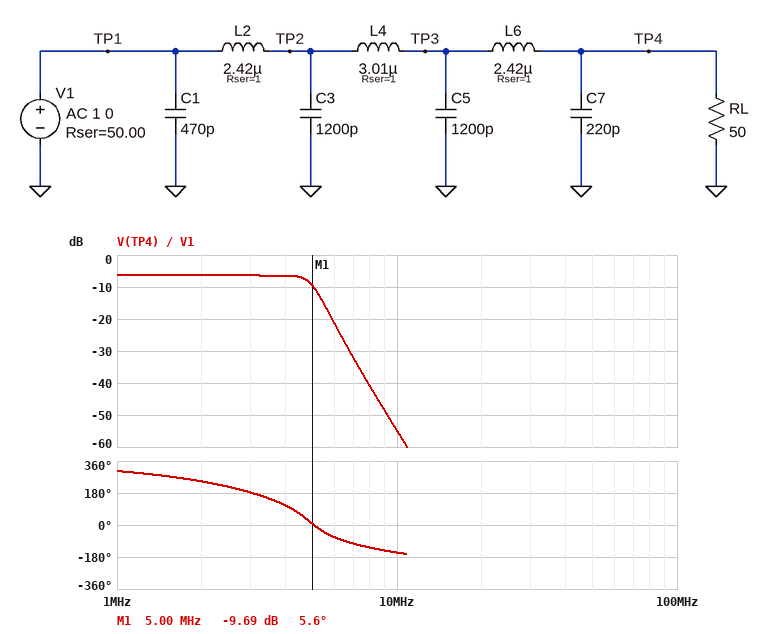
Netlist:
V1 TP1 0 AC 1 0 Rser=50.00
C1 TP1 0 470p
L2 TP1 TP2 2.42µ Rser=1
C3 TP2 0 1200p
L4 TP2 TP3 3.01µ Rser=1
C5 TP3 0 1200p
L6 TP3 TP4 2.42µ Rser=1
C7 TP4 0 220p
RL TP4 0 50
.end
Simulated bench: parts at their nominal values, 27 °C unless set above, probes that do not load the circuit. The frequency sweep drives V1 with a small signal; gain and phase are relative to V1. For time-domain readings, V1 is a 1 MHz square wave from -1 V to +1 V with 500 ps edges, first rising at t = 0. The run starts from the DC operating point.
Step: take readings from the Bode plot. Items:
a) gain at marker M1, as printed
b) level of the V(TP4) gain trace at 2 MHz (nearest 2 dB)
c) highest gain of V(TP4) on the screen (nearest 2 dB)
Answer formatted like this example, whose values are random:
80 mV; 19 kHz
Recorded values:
-9.69 dB; -6 dB; -6 dB
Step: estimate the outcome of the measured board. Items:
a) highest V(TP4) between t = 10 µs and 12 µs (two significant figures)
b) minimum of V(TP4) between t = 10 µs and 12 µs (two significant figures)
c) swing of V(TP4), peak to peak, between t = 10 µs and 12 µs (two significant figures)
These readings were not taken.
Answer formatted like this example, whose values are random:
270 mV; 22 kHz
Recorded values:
650 mV; -650 mV; 1.3 V
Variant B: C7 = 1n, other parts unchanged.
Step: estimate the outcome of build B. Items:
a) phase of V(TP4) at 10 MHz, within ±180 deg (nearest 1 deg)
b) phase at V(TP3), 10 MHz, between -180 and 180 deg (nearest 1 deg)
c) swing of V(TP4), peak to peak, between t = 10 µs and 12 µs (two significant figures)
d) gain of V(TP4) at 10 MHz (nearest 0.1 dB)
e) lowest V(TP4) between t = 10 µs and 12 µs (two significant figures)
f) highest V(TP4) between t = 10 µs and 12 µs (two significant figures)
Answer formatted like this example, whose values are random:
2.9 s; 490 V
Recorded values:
153 deg; -47 deg; 1.3 V; -63.8 dB; -670 mV; 670 mV
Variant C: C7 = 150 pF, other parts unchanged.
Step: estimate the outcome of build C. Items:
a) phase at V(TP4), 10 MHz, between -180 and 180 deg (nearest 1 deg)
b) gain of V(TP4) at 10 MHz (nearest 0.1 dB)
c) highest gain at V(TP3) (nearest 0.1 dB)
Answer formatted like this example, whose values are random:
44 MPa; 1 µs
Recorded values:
-143 deg; -54.5 dB; -3.1 dB
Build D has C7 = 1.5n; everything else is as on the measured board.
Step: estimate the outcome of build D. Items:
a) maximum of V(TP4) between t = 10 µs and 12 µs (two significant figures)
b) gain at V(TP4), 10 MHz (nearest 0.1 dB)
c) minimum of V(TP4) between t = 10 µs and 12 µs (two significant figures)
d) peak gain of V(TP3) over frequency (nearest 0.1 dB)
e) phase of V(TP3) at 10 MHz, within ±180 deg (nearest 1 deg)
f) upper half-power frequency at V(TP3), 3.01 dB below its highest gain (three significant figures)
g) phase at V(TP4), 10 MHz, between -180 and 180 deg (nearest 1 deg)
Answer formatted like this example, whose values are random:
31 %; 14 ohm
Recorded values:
640 mV; -67.4 dB; -640 mV; 1.4 dB; -47 deg; 5.16 MHz; 146 deg
